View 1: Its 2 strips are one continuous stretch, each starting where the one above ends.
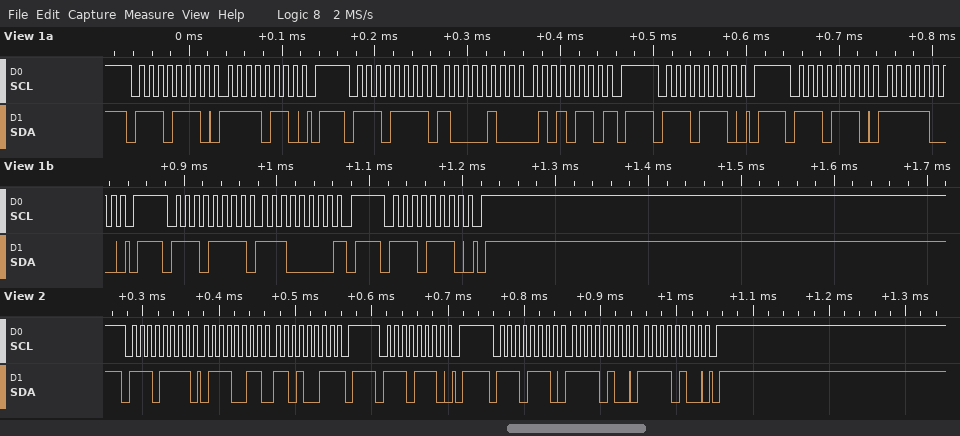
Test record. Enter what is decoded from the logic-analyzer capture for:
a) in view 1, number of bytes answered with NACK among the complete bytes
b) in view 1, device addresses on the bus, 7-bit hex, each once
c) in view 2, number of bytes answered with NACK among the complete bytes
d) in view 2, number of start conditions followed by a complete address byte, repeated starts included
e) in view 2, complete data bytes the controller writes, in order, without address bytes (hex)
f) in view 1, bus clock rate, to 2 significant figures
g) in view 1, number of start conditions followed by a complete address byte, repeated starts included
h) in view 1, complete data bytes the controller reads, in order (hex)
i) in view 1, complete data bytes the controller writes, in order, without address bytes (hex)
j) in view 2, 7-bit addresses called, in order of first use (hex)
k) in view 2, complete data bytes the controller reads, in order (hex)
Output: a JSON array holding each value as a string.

["2", "0x77", "1", "3", "F4 F4", "100 kHz", "6", "84 56 E0", "F6 F8", "0x77", "73 D3"]
